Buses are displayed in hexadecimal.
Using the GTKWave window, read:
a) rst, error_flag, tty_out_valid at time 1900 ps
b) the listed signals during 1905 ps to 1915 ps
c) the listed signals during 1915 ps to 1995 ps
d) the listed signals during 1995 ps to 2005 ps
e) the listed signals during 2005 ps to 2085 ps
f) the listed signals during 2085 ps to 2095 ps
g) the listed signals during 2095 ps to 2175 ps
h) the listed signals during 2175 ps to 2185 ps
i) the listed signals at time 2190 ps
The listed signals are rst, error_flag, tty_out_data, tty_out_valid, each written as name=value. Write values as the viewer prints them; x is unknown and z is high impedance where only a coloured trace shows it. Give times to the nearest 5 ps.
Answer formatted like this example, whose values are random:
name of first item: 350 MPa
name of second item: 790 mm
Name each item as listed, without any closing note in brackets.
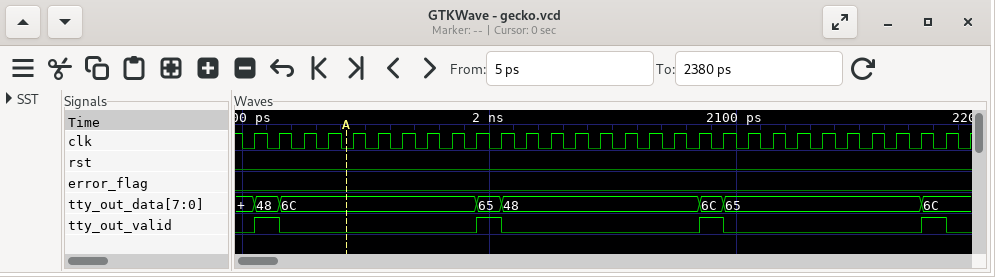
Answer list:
rst, error_flag, tty_out_valid at time 1900 ps: rst=0, error_flag=0, tty_out_valid=0
the listed signals during 1905 ps to 1915 ps: rst=0, error_flag=0, tty_out_data=48, tty_out_valid=1
the listed signals during 1915 ps to 1995 ps: rst=0, error_flag=0, tty_out_data=6C, tty_out_valid=0
the listed signals during 1995 ps to 2005 ps: rst=0, error_flag=0, tty_out_data=65, tty_out_valid=1
the listed signals during 2005 ps to 2085 ps: rst=0, error_flag=0, tty_out_data=48, tty_out_valid=0
the listed signals during 2085 ps to 2095 ps: rst=0, error_flag=0, tty_out_data=6C, tty_out_valid=1
the listed signals during 2095 ps to 2175 ps: rst=0, error_flag=0, tty_out_data=65, tty_out_valid=0
the listed signals during 2175 ps to 2185 ps: rst=0, error_flag=0, tty_out_data=6C, tty_out_valid=1
the listed signals at time 2190 ps: rst=0, error_flag=0, tty_out_data=6C, tty_out_valid=0
